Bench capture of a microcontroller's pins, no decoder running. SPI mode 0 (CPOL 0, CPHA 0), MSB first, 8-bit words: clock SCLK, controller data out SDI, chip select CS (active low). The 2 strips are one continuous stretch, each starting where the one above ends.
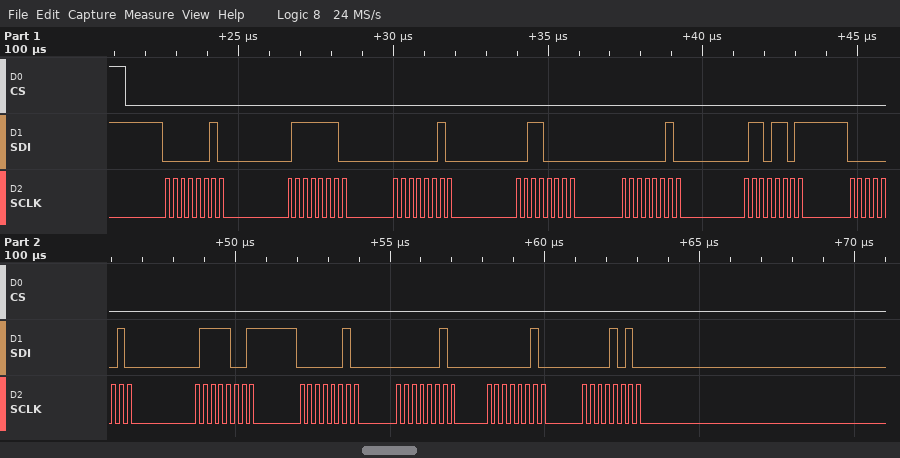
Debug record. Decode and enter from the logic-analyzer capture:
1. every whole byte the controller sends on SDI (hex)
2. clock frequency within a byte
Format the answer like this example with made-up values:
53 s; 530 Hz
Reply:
02 7E 02 30 02 6D 02 79 02 02 02 0A; 4 MHz
